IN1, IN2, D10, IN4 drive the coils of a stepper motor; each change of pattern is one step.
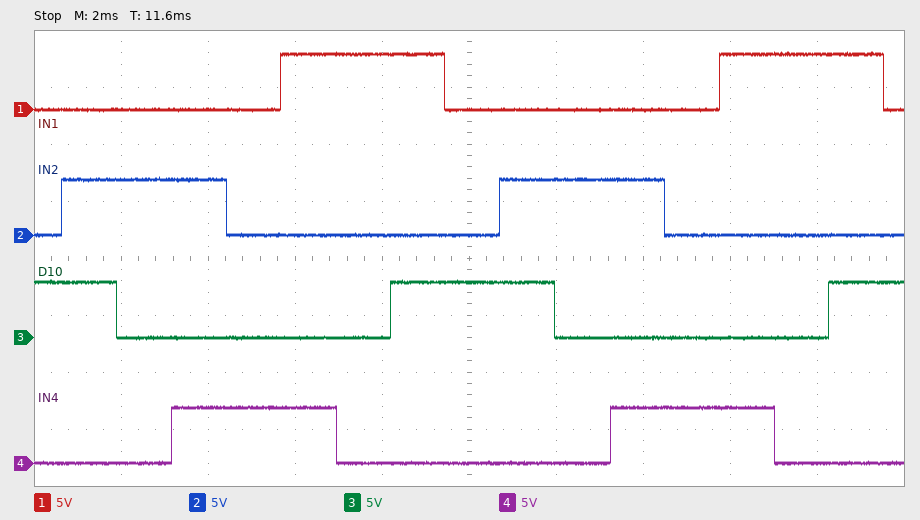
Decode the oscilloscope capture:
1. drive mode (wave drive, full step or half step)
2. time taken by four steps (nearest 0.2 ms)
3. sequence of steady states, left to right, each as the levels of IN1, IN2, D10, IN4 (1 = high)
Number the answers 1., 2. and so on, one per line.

1. half step
2. 5.0 ms
3. 0010 0110 0100 0101 0001 1001 1000 1010 0010 0110 0100 0101 0001 1001 1000 1010 0010
